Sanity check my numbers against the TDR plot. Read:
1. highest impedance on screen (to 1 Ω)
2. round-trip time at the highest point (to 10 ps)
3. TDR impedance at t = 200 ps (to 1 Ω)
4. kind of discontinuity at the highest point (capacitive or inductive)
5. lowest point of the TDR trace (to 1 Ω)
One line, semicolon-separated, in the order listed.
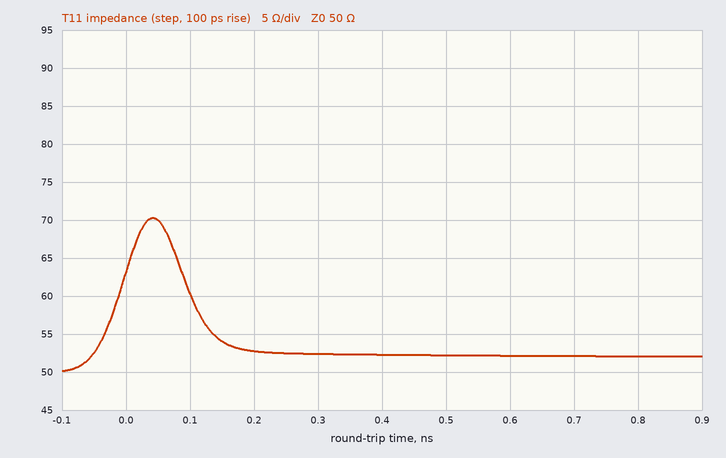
70 Ω; 40 ps; 53 Ω; inductive; 50 Ω
